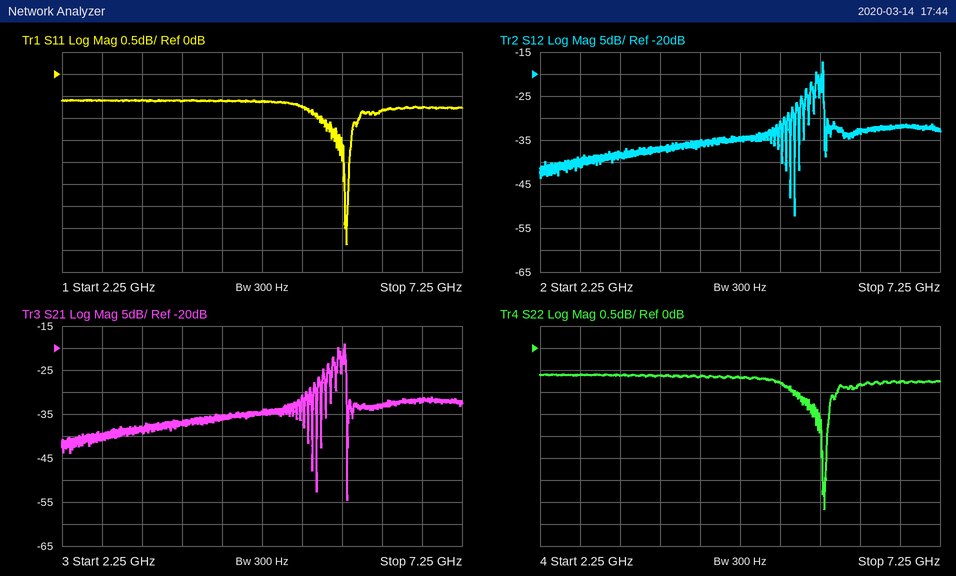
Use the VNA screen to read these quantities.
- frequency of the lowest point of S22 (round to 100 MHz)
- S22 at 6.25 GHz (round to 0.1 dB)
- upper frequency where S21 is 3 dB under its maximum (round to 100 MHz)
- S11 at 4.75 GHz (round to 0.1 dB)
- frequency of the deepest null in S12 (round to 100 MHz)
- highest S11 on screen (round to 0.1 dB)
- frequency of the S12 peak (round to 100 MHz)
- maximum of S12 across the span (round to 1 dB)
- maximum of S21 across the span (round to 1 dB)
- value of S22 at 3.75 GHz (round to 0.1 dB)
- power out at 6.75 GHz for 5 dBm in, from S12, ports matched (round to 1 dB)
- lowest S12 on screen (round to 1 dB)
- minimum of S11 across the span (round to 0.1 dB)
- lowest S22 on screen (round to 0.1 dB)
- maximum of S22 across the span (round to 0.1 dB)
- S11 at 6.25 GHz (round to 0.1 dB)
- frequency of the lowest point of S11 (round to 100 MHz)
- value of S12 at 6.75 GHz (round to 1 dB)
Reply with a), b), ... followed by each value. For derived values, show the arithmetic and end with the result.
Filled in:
a) 5.8 GHz
b) -0.8 dB
c) 5.8 GHz
d) -0.6 dB
e) 5.4 GHz
f) -0.6 dB
g) 5.8 GHz
h) -17 dB
i) -19 dB
j) -0.6 dB
k) 5 dBm + (-32 dB) = -27 dBm
l) -52 dB
m) -3.9 dB
n) -3.7 dB
o) -0.6 dB
p) -0.8 dB
q) 5.8 GHz
r) -32 dB
